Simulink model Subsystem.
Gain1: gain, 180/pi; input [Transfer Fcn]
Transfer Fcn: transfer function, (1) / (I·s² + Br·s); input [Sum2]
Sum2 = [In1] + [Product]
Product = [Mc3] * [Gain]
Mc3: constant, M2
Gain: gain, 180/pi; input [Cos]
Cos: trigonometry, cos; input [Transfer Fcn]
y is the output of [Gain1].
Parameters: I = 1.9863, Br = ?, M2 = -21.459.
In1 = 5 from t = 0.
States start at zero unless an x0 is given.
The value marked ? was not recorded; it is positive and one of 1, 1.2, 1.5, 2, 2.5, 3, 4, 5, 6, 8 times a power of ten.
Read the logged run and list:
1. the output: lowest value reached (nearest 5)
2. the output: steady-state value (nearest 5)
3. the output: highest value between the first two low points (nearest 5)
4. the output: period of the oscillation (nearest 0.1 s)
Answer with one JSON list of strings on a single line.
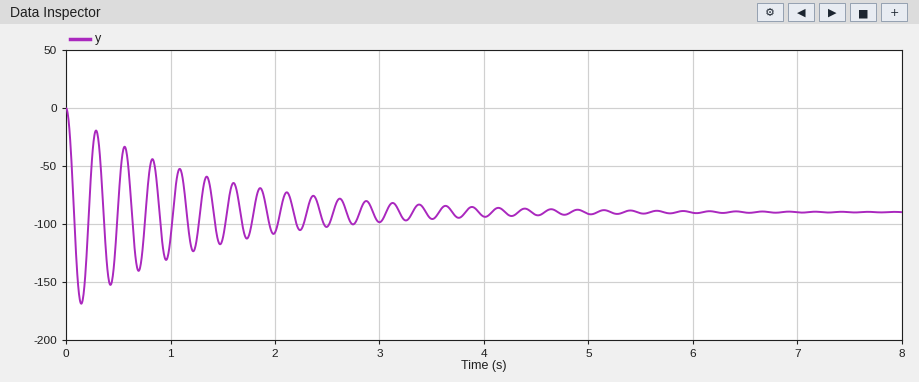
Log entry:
["-170", "-90", "-20", "0.3 s"]
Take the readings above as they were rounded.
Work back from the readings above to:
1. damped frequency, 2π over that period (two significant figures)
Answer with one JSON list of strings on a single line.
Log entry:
["21 rad/s"]
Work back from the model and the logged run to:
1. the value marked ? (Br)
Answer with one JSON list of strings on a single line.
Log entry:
["3"]
